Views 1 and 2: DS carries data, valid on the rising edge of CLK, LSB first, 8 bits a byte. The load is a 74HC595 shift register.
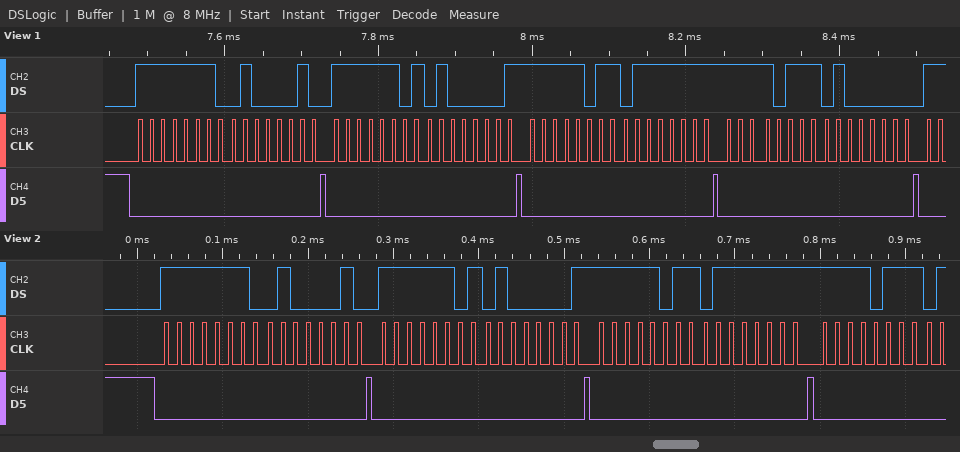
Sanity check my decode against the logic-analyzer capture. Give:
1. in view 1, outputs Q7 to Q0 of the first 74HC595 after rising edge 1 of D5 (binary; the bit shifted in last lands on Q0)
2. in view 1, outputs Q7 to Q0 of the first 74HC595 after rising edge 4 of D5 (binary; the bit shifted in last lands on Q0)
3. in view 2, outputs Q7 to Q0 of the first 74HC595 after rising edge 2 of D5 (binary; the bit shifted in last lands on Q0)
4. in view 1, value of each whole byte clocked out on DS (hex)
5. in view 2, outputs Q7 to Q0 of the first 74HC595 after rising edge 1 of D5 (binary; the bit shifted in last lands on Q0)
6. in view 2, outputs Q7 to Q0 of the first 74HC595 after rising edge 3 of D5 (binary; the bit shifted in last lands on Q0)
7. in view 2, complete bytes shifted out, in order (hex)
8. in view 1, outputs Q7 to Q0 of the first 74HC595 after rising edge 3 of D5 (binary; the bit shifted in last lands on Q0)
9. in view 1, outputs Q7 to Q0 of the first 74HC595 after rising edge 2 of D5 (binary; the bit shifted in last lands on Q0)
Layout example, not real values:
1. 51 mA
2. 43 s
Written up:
1. 01000010
2. 01000000
3. 01000001
4. 0x7F 0x42 0xBF 0x82 0xDF 0xFE 0xEF 0x02
5. 01000010
6. 01111111
7. 7F 42 BF 82 DF FE EF
8. 01111111
9. 01000001
